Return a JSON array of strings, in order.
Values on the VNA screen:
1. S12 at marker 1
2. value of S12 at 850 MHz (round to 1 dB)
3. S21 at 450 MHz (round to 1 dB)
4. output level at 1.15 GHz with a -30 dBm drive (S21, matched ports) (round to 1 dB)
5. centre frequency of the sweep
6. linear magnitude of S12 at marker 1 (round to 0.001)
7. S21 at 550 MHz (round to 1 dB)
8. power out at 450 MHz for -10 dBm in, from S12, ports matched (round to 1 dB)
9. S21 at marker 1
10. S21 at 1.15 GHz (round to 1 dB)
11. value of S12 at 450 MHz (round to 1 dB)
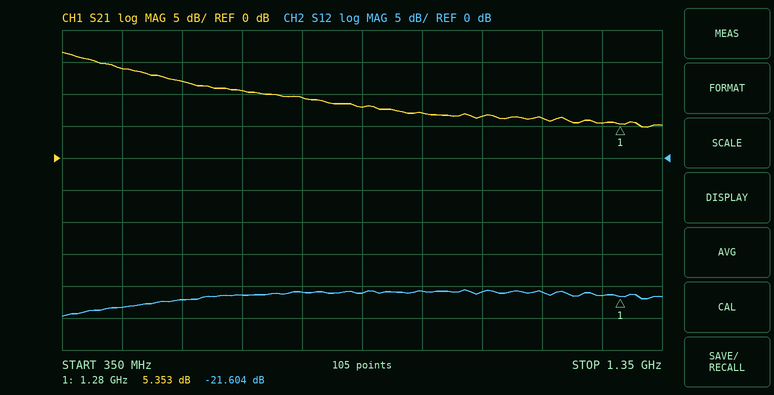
["-21.604 dB", "-21 dB", "14 dB", "-24 dBm", "850 MHz", "0.083", "12 dB", "-33 dBm", "5.353 dB", "6 dB", "-23 dB"]
